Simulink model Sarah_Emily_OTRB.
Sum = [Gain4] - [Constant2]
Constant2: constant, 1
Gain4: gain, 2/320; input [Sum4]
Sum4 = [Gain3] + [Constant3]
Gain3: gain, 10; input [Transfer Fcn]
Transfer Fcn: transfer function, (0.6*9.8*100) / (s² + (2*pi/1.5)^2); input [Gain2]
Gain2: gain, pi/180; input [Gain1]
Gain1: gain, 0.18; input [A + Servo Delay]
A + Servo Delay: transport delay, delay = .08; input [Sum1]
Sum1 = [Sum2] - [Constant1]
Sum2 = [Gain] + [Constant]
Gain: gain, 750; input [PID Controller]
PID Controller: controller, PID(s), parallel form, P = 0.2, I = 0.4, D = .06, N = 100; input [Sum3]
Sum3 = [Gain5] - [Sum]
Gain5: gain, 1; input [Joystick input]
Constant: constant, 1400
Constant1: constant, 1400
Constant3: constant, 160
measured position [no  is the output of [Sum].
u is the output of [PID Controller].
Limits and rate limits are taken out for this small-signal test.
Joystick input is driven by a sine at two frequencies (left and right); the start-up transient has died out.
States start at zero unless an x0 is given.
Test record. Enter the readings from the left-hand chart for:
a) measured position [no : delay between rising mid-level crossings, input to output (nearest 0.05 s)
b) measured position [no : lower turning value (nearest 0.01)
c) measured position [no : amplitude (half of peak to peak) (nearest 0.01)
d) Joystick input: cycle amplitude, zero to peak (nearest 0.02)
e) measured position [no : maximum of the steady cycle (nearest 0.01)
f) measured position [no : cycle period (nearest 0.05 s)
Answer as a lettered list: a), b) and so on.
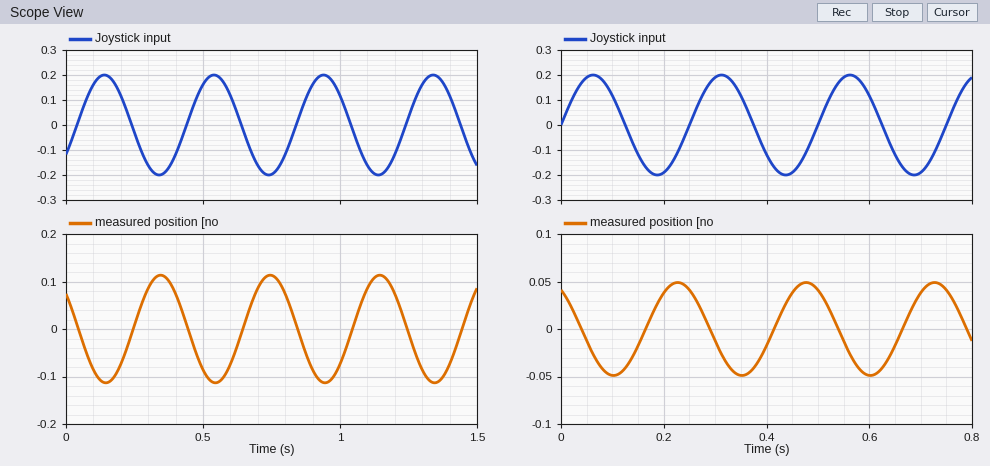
a) 0.20 s
b) -0.11
c) 0.11
d) 0.20
e) 0.11
f) 0.40 s
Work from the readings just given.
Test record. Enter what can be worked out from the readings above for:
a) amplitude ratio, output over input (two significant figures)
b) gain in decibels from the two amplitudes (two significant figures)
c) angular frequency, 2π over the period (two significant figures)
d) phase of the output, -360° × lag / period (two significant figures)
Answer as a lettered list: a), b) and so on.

a) 0.55
b) -5.2 dB
c) 16 rad/s
d) -180°
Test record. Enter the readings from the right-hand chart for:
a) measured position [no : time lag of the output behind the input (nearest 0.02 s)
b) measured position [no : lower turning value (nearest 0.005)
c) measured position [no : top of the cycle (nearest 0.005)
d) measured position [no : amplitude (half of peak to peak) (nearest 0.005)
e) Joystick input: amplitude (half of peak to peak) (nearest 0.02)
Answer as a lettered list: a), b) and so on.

a) 0.16 s
b) -0.050
c) 0.050
d) 0.050
e) 0.20
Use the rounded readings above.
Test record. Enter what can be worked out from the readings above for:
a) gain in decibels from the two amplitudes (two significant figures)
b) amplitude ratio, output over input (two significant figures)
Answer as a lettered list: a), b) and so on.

a) -12 dB
b) 0.25
